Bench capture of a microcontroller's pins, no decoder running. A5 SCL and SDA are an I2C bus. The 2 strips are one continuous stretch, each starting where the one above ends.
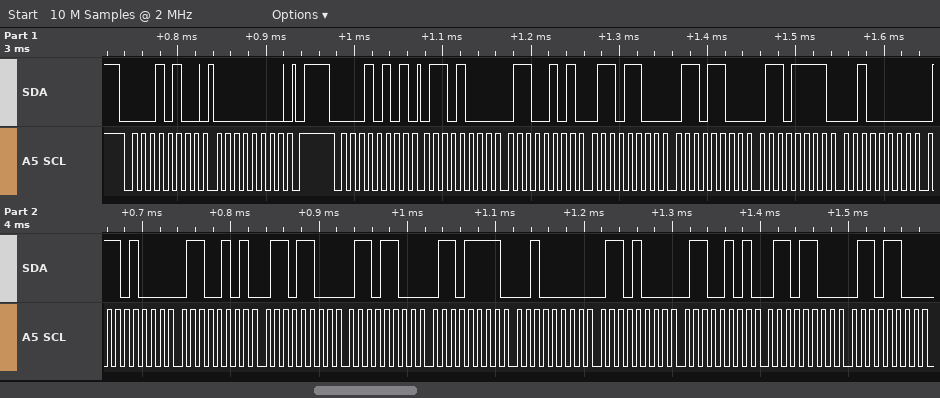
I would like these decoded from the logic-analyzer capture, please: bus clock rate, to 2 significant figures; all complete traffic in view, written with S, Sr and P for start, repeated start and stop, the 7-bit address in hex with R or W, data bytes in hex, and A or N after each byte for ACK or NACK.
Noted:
100 kHz
S 0AW A 00 A P S 0AR A 68 A 65 A 6C A 6C A 6F A 20 A 68 A 65 A 6C A 6C A 6F A 20 A 68 A 65 A 6C A 6C A
